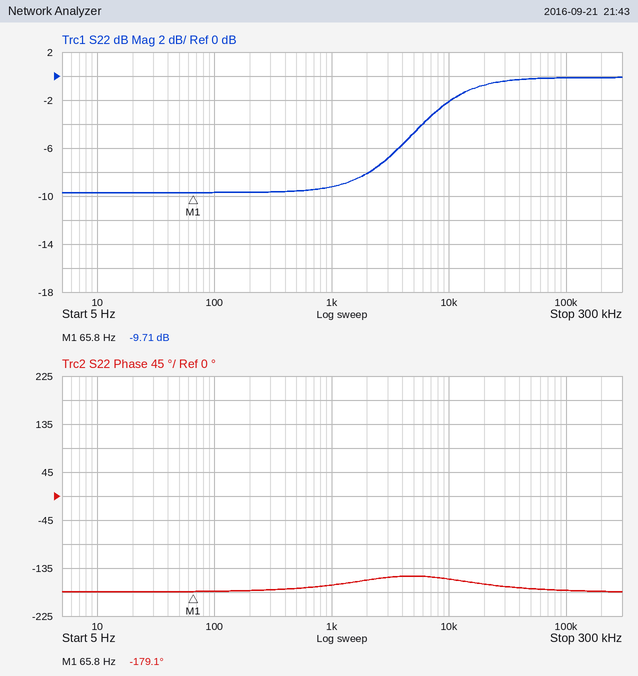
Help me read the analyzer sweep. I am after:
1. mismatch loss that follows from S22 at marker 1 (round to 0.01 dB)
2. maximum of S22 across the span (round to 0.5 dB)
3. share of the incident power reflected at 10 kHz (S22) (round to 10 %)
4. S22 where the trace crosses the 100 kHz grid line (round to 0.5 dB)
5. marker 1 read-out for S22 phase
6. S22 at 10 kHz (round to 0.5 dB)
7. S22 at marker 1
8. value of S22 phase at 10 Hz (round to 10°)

0.49 dB
0.0 dB
60 %
0.0 dB
-179.1°
-2.0 dB
-9.71 dB
-180°
